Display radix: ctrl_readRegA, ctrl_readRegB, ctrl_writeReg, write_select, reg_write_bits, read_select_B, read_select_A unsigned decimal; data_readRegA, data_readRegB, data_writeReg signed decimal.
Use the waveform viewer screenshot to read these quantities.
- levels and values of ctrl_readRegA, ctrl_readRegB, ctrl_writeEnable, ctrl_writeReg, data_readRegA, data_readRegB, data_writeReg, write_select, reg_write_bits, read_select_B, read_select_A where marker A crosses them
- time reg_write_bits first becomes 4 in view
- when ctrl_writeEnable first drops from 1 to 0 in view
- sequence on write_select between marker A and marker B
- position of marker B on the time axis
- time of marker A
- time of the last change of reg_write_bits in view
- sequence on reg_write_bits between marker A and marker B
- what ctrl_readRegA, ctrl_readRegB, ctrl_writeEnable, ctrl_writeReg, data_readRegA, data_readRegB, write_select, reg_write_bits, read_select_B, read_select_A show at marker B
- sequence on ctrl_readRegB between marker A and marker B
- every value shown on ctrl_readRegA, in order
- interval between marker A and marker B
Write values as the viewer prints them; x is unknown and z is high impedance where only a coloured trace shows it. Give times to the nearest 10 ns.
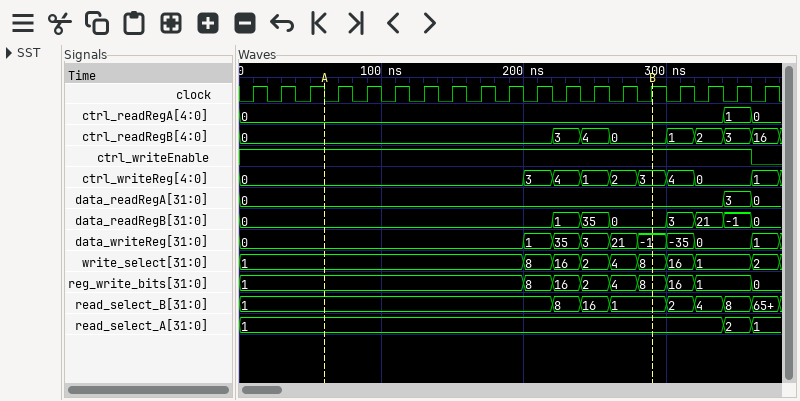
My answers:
ctrl_readRegA=0, ctrl_readRegB=0, ctrl_writeEnable=1, ctrl_writeReg=0, data_readRegA=0, data_readRegB=0, data_writeReg=0, write_select=1, reg_write_bits=1, read_select_B=1, read_select_A=1
260 ns
360 ns
1, 8, 16, 2, 4, 8
290 ns
60 ns
360 ns
1, 8, 16, 2, 4, 8
ctrl_readRegA=0, ctrl_readRegB=0, ctrl_writeEnable=1, ctrl_writeReg=3, data_readRegA=0, data_readRegB=0, write_select=8, reg_write_bits=8, read_select_B=1, read_select_A=1
0, 3, 4, 0
0, 1, 0
230 ns
